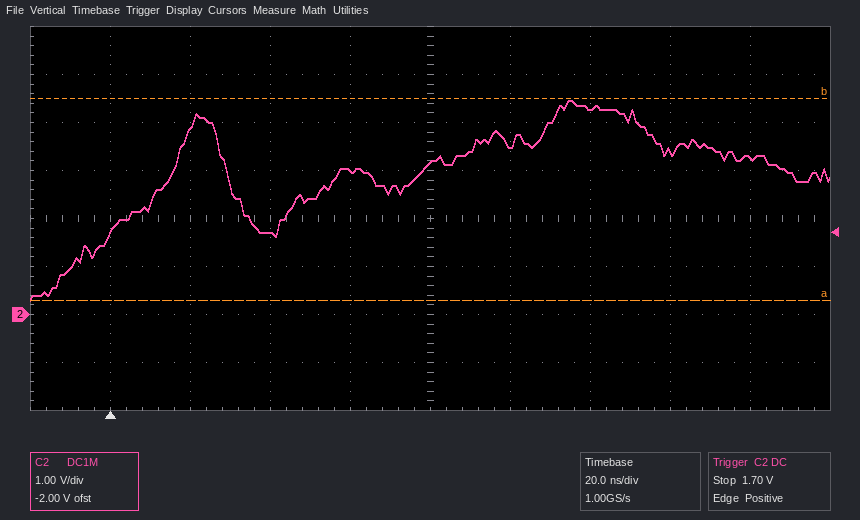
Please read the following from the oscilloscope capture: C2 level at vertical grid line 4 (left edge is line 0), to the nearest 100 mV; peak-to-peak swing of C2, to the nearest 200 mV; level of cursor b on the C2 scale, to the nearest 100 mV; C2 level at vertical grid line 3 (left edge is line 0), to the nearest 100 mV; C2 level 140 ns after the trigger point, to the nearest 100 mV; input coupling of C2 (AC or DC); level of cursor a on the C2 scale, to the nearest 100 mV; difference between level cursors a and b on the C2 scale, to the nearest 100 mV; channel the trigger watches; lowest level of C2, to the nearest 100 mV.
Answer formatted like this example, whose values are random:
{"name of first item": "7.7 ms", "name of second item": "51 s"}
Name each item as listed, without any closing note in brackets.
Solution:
{"C2 level at vertical grid line 4 (left edge is line 0), to the nearest 100 mV": "3.0 V", "peak-to-peak swing of C2, to the nearest 200 mV": "4.2 V", "level of cursor b on the C2 scale, to the nearest 100 mV": "4.5 V", "C2 level at vertical grid line 3 (left edge is line 0), to the nearest 100 mV": "1.7 V", "C2 level 140 ns after the trigger point, to the nearest 100 mV": "3.4 V", "input coupling of C2": "DC", "level of cursor a on the C2 scale, to the nearest 100 mV": "300 mV", "difference between level cursors a and b on the C2 scale, to the nearest 100 mV": "4.2 V", "channel the trigger watches": "C2", "lowest level of C2, to the nearest 100 mV": "300 mV"}
